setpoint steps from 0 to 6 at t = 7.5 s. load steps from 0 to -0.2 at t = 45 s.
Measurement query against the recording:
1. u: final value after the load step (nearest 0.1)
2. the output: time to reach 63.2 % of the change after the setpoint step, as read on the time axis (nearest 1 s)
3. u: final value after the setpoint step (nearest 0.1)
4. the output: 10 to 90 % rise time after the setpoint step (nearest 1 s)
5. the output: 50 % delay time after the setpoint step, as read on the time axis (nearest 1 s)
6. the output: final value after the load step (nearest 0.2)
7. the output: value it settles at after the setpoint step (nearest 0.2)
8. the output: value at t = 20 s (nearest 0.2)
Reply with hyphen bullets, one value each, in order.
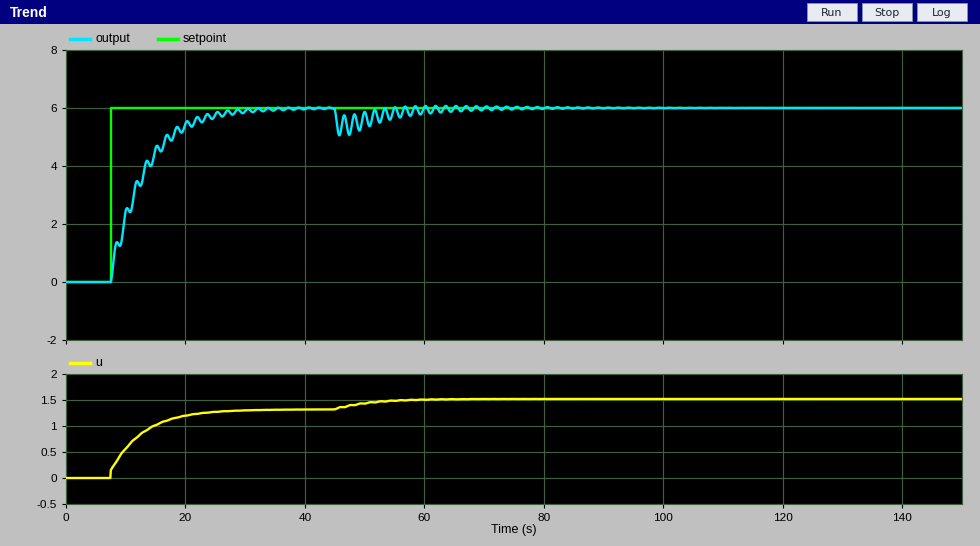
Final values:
- 1.5
- 13 s
- 1.3
- 12 s
- 11 s
- 6.0
- 6.0
- 5.4
